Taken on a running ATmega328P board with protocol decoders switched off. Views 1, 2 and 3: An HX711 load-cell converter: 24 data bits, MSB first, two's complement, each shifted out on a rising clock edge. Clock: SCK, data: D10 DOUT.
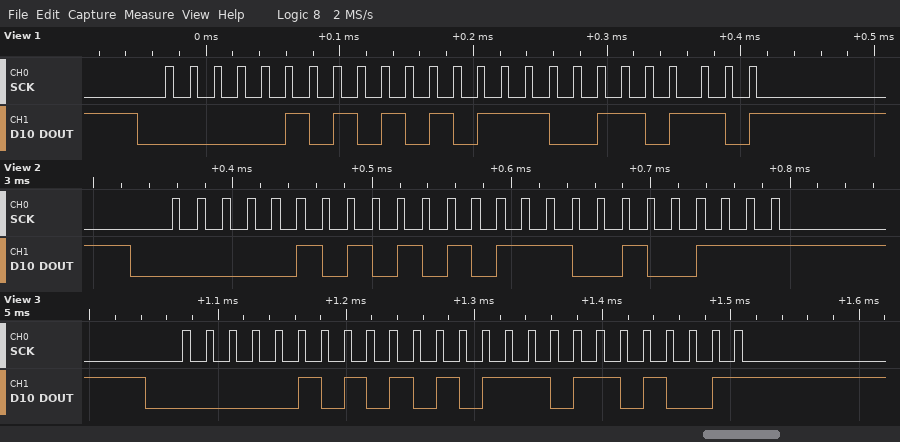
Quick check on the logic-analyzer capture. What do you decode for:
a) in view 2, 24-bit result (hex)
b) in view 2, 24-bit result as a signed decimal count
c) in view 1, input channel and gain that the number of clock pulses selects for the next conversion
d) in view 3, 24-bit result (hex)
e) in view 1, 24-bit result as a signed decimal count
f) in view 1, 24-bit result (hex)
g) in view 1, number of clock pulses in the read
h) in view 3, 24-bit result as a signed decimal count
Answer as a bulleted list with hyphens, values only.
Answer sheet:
- 0x055727
- 349991
- channel A, gain 128
- 0x055769
- 350006
- 0x055736
- 25
- 350057
